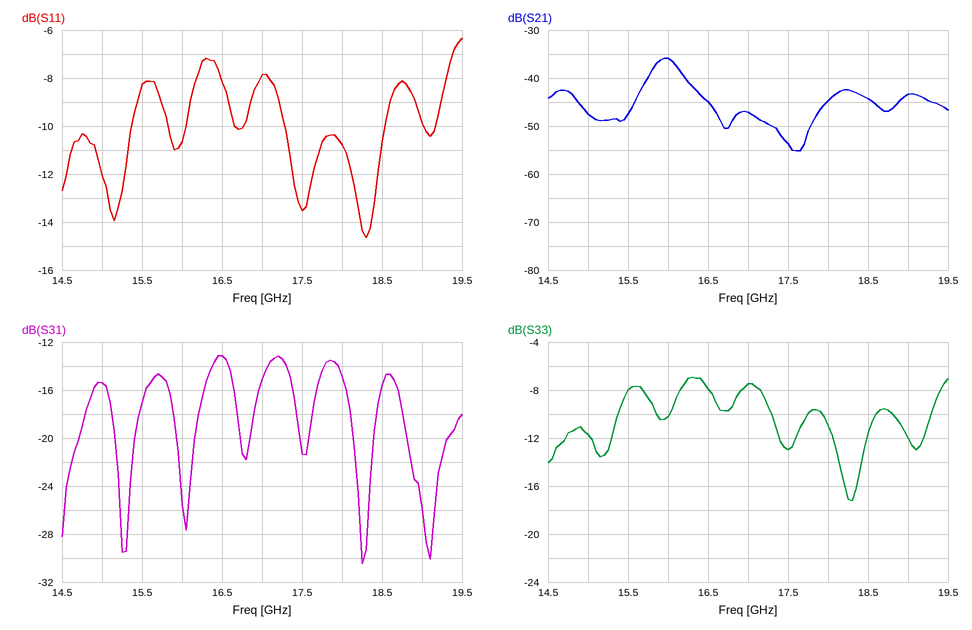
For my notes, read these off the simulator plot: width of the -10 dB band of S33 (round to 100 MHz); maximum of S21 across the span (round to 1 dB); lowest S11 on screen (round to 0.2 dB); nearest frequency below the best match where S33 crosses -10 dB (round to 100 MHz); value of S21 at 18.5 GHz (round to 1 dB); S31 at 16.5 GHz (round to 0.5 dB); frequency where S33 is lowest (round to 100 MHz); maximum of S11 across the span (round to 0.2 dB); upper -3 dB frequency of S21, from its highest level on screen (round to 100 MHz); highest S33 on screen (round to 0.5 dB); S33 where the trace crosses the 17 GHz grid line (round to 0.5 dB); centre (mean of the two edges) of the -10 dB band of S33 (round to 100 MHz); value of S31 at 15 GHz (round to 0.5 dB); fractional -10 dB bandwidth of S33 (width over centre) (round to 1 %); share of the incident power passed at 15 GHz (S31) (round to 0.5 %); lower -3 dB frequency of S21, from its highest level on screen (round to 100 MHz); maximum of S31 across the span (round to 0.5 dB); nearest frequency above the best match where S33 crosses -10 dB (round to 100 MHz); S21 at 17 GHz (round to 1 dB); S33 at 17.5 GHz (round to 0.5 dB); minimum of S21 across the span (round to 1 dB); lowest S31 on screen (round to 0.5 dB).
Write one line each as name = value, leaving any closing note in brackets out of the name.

width of the -10 dB band of S33 = 700 MHz
maximum of S21 across the span = -36 dB
lowest S11 on screen = -14.6 dB
nearest frequency below the best match where S33 crosses -10 dB = 17.9 GHz
value of S21 at 18.5 GHz = -44 dB
S31 at 16.5 GHz = -13.0 dB
frequency where S33 is lowest = 18.3 GHz
maximum of S11 across the span = -6.4 dB
upper -3 dB frequency of S21, from its highest level on screen = 16.2 GHz
highest S33 on screen = -7.0 dB
S33 where the trace crosses the 17 GHz grid line = -7.5 dB
centre (mean of the two edges) of the -10 dB band of S33 = 18.3 GHz
value of S31 at 15 GHz = -15.5 dB
fractional -10 dB bandwidth of S33 (width over centre) = 4 %
share of the incident power passed at 15 GHz (S31) = 3.0 %
lower -3 dB frequency of S21, from its highest level on screen = 15.8 GHz
maximum of S31 across the span = -13.0 dB
nearest frequency above the best match where S33 crosses -10 dB = 18.6 GHz
S21 at 17 GHz = -47 dB
S33 at 17.5 GHz = -13.0 dB
minimum of S21 across the span = -55 dB
lowest S31 on screen = -30.5 dB
